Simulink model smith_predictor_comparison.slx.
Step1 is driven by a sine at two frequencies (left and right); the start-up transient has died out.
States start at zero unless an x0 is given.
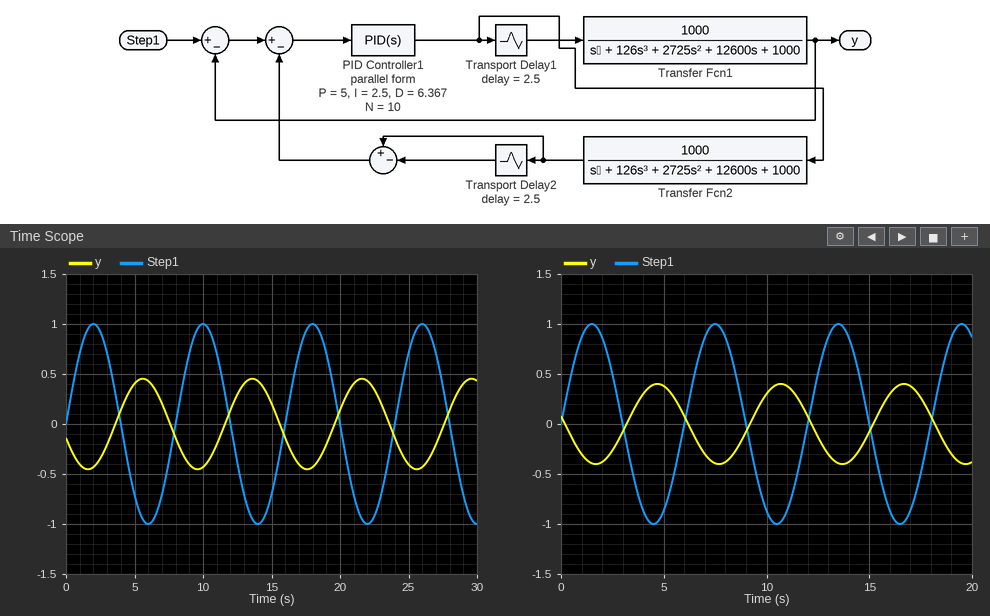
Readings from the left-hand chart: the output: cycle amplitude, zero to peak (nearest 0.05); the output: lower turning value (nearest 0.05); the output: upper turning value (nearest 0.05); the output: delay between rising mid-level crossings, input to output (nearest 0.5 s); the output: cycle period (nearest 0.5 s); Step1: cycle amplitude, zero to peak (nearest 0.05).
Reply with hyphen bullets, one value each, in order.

- 0.45
- -0.45
- 0.45
- 3.5 s
- 8.0 s
- 1.00
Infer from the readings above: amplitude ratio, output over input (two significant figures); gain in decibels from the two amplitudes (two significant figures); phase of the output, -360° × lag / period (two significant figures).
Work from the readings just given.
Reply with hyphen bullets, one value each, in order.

- 0.45
- -6.9 dB
- -160°
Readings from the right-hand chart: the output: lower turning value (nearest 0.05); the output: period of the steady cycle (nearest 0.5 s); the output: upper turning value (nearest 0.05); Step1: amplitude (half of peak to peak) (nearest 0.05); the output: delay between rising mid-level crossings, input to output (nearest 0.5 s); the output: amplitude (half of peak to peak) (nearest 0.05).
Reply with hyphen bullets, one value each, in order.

- -0.40
- 6.0 s
- 0.40
- 1.00
- 3.0 s
- 0.40
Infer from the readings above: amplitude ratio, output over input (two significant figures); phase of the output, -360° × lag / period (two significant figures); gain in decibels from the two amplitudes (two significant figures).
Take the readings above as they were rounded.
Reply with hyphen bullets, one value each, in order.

- 0.40
- -180°
- -8.0 dB
